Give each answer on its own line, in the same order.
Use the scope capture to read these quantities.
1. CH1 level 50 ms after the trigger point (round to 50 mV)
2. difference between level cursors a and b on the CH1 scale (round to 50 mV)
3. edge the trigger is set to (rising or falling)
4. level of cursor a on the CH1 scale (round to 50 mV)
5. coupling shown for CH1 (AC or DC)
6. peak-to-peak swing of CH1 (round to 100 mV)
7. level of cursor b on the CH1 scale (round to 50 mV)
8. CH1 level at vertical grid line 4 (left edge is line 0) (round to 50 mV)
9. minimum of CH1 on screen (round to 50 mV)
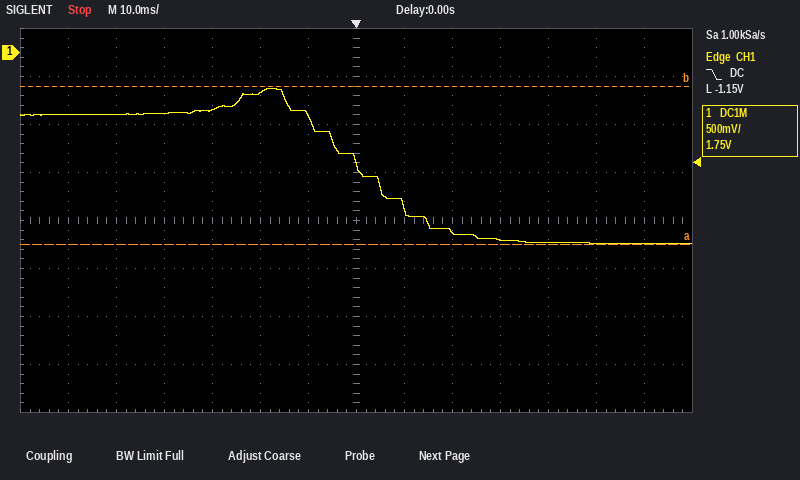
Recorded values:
-2.00 V
1.65 V
falling
-2.00 V
DC
1.60 V
-350 mV
-600 mV
-2.00 V
